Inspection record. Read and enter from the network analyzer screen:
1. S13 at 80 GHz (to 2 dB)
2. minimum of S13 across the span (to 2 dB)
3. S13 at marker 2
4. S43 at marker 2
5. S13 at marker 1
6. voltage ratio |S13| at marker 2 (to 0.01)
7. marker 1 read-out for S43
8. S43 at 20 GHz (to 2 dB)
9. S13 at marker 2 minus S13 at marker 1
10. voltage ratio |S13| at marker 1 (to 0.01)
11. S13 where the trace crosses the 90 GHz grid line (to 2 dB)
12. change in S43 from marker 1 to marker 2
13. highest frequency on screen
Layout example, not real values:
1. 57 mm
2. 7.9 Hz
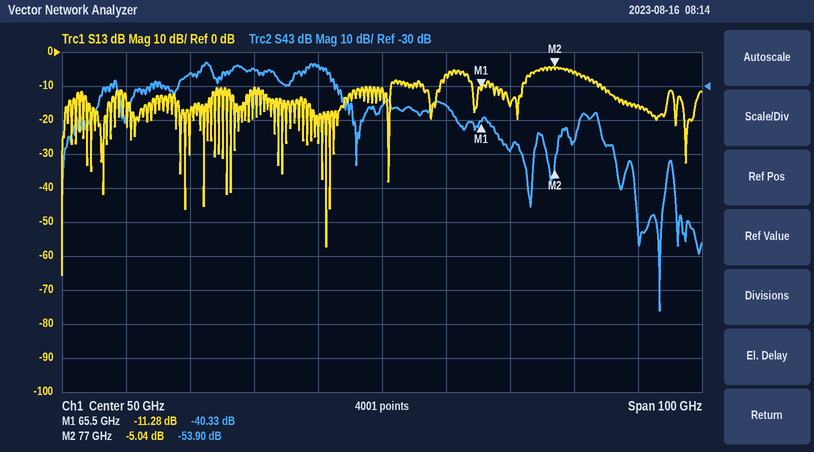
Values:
1. -6 dB
2. -66 dB
3. -5.04 dB
4. -53.90 dB
5. -11.28 dB
6. 0.56
7. -40.33 dB
8. -26 dB
9. 6.24 dB
10. 0.27
11. -16 dB
12. -13.57 dB
13. 100 GHz
